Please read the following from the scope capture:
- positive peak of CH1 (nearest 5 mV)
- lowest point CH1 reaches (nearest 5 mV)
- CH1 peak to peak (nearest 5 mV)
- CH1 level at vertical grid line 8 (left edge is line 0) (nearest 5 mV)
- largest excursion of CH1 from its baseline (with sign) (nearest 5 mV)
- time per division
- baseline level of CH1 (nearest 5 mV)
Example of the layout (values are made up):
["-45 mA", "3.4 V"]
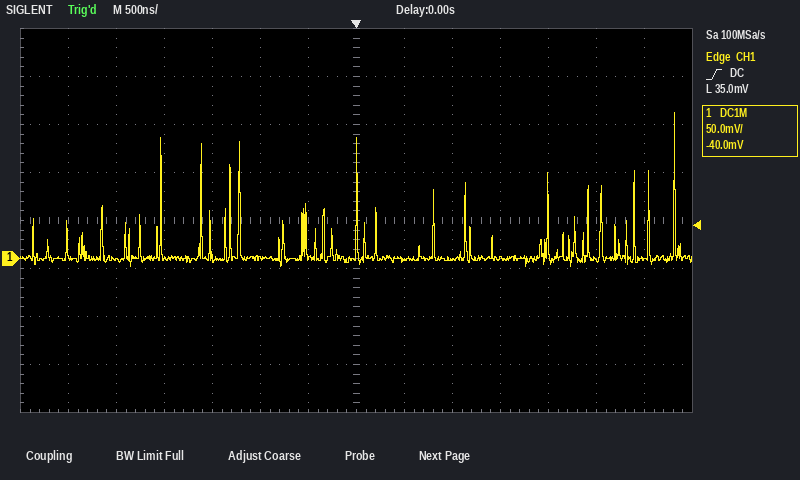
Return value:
["150 mV", "-10 mV", "160 mV", "0 mV", "+150 mV", "500 ns", "0 mV"]
